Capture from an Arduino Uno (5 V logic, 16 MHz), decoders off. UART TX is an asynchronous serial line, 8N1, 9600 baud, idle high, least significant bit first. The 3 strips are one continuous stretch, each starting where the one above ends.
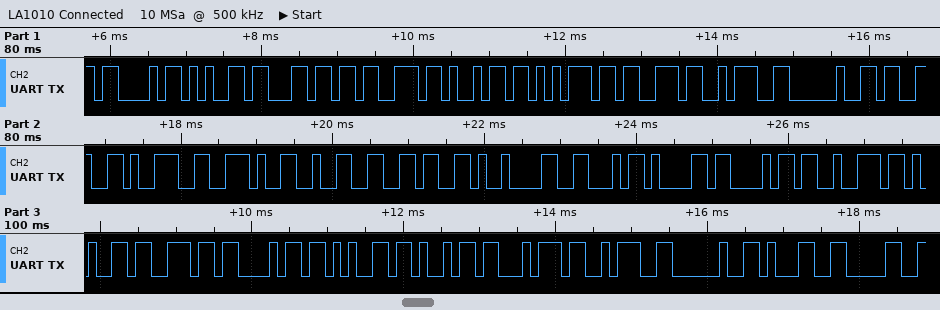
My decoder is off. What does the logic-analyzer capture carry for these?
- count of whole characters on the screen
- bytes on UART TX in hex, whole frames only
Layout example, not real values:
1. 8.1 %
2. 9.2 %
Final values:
1. 29
2. 43 65 6C 73 69 75 73 3A 20 33 39 2E 32 36 09 46 61 68 72 65 6E 68 65 69 74 3A 20 31 30
